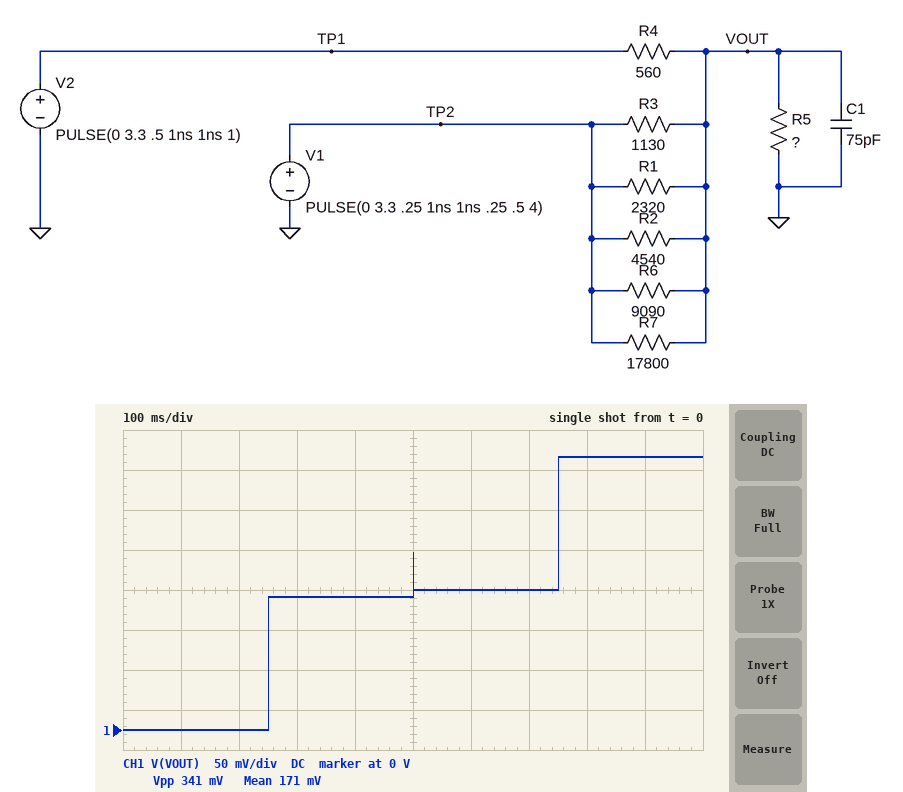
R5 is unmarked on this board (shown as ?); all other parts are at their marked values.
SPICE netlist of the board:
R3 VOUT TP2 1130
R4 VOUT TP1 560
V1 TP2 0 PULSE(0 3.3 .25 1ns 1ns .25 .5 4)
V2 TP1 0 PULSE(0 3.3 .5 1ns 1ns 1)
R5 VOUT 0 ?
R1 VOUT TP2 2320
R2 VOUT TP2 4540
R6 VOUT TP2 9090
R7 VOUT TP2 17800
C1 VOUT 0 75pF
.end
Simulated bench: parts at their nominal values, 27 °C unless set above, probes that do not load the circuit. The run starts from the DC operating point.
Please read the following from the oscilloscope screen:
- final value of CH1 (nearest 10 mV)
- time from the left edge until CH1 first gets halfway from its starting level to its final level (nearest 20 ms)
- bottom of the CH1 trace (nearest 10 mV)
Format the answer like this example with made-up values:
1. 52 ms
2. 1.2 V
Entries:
1. 340 mV
2. 500 ms
3. 0 V
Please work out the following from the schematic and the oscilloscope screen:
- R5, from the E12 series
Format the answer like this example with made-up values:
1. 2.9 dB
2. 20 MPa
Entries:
1. 33 Ω
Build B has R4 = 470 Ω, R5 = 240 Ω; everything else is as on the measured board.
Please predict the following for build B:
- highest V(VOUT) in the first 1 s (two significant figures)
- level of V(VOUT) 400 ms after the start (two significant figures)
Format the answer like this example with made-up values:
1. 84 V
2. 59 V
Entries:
1. 1.6 V
2. 700 mV
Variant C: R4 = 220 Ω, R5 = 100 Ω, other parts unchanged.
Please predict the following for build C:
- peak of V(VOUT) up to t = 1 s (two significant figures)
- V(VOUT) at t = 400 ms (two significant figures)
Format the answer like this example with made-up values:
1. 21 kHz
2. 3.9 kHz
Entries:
1. 1.3 V
2. 350 mV
